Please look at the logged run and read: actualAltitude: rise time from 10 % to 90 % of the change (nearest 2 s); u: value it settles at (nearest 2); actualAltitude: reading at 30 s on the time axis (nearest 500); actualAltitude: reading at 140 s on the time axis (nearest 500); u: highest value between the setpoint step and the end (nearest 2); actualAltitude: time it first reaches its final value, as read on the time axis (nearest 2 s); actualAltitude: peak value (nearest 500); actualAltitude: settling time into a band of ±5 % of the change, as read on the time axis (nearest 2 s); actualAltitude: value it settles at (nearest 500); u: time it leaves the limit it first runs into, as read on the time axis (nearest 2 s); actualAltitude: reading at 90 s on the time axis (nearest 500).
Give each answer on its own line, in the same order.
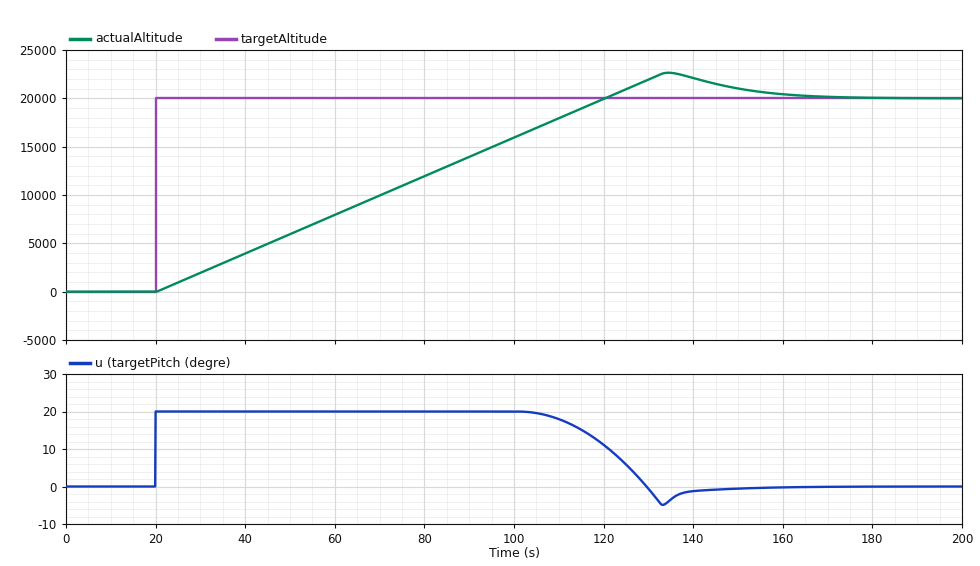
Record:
80 s
0
2000
22000
20
120 s
22500
150 s
20000
104 s
14000
